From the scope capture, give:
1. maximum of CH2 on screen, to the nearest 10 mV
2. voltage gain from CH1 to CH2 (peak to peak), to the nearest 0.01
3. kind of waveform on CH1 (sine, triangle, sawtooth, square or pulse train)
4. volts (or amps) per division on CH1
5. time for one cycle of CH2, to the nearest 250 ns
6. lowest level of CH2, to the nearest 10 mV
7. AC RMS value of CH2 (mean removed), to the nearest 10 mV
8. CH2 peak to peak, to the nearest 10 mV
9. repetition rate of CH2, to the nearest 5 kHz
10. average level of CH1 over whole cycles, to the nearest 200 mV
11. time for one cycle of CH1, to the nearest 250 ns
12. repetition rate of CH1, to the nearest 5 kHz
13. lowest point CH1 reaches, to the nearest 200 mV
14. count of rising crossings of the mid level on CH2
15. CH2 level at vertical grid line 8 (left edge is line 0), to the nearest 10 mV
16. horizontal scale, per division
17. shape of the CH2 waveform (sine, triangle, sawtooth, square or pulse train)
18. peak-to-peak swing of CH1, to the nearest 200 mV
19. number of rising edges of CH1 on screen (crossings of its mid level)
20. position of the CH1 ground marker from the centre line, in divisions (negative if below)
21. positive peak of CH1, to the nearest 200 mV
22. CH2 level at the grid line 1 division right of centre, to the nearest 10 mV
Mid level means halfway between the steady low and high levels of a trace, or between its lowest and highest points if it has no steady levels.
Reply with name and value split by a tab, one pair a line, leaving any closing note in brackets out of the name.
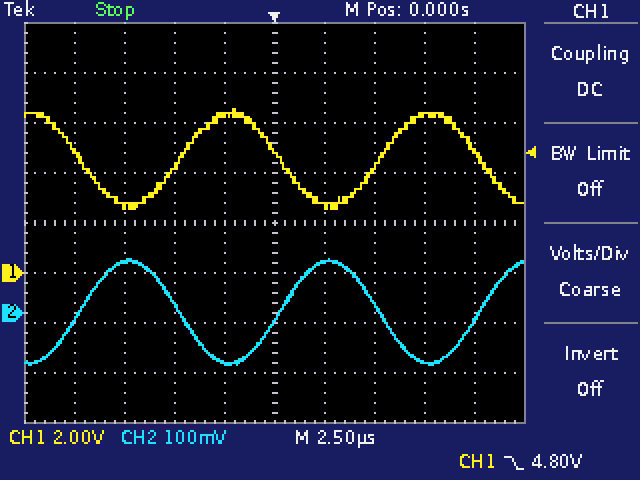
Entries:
maximum of CH2 on screen, to the nearest 10 mV	110 mV
voltage gain from CH1 to CH2 (peak to peak), to the nearest 0.01	0.05
kind of waveform on CH1	sine
volts (or amps) per division on CH1	2 V
time for one cycle of CH2, to the nearest 250 ns	10.00 µs
lowest level of CH2, to the nearest 10 mV	-100 mV
AC RMS value of CH2 (mean removed), to the nearest 10 mV	70 mV
CH2 peak to peak, to the nearest 10 mV	210 mV
repetition rate of CH2, to the nearest 5 kHz	100 kHz
average level of CH1 over whole cycles, to the nearest 200 mV	4.6 V
time for one cycle of CH1, to the nearest 250 ns	10.00 µs
repetition rate of CH1, to the nearest 5 kHz	100 kHz
lowest point CH1 reaches, to the nearest 200 mV	2.6 V
count of rising crossings of the mid level on CH2	3
CH2 level at vertical grid line 8 (left edge is line 0), to the nearest 10 mV	-100 mV
horizontal scale, per division	2.5 µs
shape of the CH2 waveform	sine
peak-to-peak swing of CH1, to the nearest 200 mV	4.0 V
number of rising edges of CH1 on screen	2
position of the CH1 ground marker from the centre line, in divisions	-1.0 div
positive peak of CH1, to the nearest 200 mV	6.6 V
CH2 level at the grid line 1 division right of centre, to the nearest 10 mV	100 mV
